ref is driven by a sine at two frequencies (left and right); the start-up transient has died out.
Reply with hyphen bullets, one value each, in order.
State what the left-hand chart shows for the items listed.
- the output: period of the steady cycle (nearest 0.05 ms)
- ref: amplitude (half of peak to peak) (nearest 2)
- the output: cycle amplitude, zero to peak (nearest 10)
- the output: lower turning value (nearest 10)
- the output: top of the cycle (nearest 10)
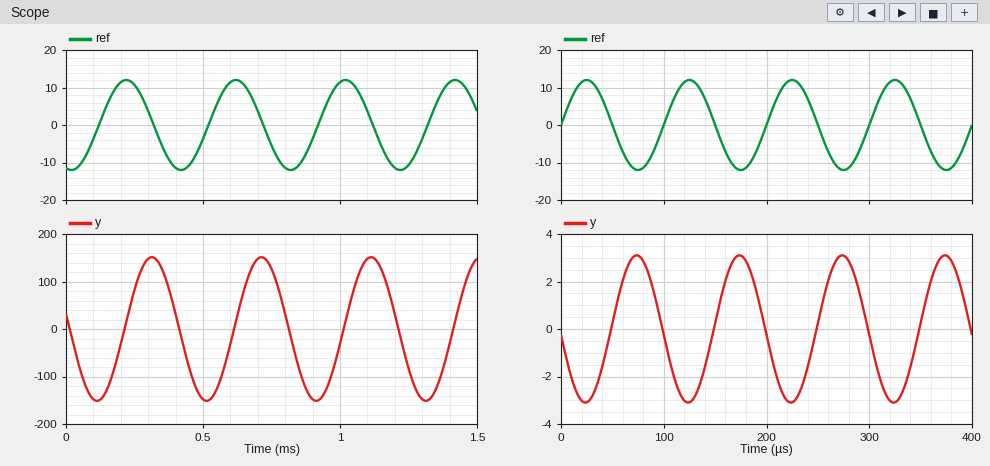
- 0.40 ms
- 12
- 150
- -150
- 150
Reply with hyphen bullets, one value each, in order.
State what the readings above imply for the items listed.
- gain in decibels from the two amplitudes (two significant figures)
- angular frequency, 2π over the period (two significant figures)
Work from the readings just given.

- 22 dB
- 16 rad/ms
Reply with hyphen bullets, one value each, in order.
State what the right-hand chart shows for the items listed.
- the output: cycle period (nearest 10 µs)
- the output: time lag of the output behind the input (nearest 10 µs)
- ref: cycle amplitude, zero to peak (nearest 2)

- 100 µs
- 50 µs
- 12
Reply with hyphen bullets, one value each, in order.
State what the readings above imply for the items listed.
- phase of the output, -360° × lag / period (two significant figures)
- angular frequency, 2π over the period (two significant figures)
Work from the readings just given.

- -180°
- 0.063 rad/µs
